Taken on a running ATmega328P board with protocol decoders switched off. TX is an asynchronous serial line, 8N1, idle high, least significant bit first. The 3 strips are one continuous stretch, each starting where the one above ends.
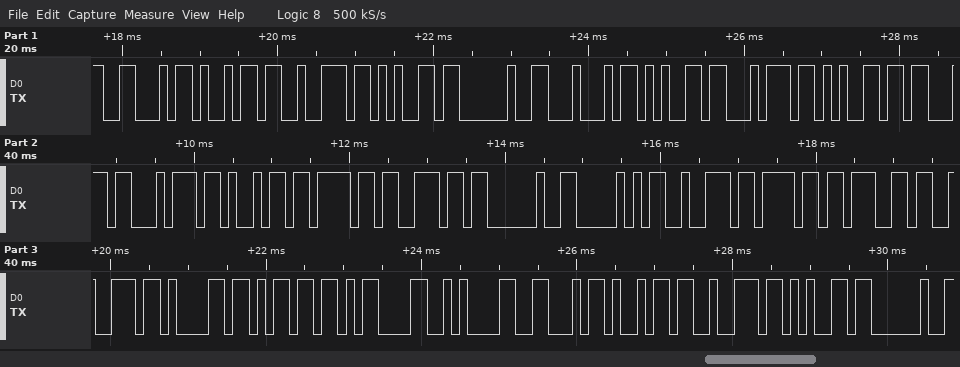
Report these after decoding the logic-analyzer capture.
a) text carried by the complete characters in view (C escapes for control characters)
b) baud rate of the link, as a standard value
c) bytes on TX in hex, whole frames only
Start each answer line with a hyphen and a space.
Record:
- "Fire Detection Program\r\nFire "
- 9600 baud
- 0x46 0x69 0x72 0x65 0x20 0x44 0x65 0x74 0x65 0x63 0x74 0x69 0x6F 0x6E 0x20 0x50 0x72 0x6F 0x67 0x72 0x61 0x6D 0x0D 0x0A 0x46 0x69 0x72 0x65 0x20
